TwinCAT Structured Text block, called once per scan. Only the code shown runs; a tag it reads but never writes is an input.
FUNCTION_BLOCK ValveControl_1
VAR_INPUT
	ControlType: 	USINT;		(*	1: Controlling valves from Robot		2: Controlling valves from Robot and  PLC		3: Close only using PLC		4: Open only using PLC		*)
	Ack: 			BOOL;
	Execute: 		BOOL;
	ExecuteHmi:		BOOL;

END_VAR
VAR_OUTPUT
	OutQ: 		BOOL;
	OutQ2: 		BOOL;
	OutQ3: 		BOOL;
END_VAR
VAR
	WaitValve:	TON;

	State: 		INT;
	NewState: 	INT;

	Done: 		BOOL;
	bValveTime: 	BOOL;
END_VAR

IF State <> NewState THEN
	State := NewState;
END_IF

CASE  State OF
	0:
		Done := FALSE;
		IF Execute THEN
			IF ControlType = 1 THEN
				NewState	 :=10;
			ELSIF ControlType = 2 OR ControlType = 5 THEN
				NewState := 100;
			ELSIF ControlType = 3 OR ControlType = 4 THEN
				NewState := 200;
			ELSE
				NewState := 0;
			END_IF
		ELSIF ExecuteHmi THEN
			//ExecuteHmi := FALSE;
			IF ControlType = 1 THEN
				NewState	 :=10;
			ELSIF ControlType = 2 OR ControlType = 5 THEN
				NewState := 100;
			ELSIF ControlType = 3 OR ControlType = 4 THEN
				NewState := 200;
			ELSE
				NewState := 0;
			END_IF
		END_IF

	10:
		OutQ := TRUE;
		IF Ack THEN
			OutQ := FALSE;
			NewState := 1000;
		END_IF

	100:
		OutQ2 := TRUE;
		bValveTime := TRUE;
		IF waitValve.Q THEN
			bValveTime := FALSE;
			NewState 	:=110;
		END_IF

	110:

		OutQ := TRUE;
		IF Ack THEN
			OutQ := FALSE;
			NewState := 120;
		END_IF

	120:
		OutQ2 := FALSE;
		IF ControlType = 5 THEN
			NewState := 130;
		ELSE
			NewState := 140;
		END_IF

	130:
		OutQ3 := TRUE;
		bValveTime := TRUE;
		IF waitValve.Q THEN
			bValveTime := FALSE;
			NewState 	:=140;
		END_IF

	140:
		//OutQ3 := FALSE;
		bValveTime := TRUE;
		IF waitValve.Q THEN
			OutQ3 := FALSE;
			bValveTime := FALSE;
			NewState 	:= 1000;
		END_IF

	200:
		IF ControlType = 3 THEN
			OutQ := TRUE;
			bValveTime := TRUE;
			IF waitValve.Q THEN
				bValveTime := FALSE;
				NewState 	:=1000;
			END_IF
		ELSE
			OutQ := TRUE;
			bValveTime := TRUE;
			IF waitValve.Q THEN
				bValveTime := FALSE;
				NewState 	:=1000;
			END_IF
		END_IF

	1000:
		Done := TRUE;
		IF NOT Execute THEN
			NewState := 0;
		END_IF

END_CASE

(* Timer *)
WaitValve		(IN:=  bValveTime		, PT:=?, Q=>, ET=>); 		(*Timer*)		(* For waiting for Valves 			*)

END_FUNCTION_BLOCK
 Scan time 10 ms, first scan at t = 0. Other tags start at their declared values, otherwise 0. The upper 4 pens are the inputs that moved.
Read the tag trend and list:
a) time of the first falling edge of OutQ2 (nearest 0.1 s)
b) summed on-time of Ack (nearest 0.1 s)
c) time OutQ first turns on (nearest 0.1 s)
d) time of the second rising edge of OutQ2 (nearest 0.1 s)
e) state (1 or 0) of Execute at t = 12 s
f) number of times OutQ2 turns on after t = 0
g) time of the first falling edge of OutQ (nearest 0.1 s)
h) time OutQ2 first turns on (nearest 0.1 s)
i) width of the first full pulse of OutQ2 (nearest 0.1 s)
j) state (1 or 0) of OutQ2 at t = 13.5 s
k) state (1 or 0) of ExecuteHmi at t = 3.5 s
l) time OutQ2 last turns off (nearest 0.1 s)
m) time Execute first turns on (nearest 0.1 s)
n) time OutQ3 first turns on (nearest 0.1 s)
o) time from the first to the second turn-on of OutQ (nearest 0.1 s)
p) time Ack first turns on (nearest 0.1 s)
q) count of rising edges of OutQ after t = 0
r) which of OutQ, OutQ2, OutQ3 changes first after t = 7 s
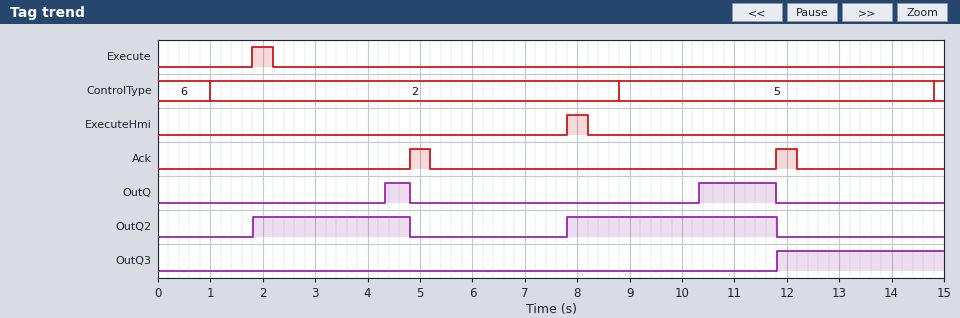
4.8 s
0.8 s
4.3 s
7.8 s
0
2
4.8 s
1.8 s
3.0 s
0
0
11.8 s
1.8 s
11.8 s
6.0 s
4.8 s
2
OutQ2
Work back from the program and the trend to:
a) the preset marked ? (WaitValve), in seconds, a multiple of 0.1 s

2.5 s
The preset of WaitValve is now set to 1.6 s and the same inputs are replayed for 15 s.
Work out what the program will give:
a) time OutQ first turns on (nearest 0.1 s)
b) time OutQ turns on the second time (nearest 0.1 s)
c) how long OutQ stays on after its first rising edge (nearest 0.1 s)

3.4 s
9.4 s
1.4 s
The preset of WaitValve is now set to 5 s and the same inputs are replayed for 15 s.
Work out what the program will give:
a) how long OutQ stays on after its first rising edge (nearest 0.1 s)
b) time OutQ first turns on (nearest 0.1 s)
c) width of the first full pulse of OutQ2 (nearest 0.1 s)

5.0 s
6.8 s
10.0 s
